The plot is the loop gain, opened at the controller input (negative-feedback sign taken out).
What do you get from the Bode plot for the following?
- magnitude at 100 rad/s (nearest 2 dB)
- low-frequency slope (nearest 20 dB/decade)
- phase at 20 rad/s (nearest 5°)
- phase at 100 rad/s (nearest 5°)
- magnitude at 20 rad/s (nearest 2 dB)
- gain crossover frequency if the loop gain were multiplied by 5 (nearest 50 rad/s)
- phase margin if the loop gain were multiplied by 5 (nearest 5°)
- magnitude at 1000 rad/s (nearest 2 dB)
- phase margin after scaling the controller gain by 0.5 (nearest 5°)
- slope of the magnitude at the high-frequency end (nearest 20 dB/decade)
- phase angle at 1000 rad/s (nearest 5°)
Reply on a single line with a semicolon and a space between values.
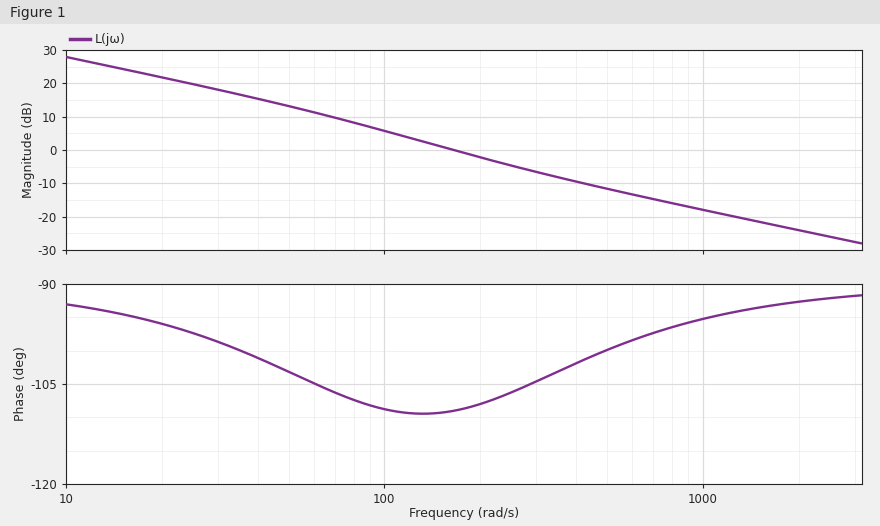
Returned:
6 dB; -20 dB/decade; -95°; -110°; 22 dB; 650 rad/s; 80°; -18 dB; 70°; -20 dB/decade; -95°
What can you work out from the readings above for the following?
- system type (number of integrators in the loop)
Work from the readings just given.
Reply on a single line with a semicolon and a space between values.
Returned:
1
